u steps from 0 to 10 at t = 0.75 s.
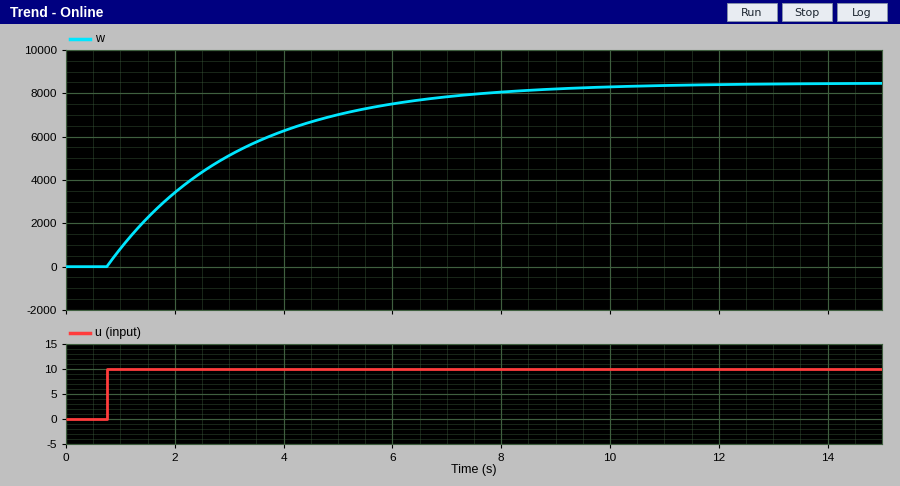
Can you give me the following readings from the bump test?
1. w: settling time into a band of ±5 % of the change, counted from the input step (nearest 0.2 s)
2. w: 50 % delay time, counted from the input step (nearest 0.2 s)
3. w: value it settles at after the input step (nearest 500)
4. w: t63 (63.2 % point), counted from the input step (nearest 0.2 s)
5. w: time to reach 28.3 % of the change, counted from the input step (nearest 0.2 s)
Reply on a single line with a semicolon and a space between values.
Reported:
7.2 s; 1.6 s; 8500; 2.4 s; 0.8 s
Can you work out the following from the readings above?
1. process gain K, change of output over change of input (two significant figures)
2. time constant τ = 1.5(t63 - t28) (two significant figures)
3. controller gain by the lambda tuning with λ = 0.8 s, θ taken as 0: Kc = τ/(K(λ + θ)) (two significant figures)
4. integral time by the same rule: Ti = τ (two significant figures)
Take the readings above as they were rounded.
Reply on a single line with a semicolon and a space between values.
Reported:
850; 2.4 s; 0.0035; 2.4 s
